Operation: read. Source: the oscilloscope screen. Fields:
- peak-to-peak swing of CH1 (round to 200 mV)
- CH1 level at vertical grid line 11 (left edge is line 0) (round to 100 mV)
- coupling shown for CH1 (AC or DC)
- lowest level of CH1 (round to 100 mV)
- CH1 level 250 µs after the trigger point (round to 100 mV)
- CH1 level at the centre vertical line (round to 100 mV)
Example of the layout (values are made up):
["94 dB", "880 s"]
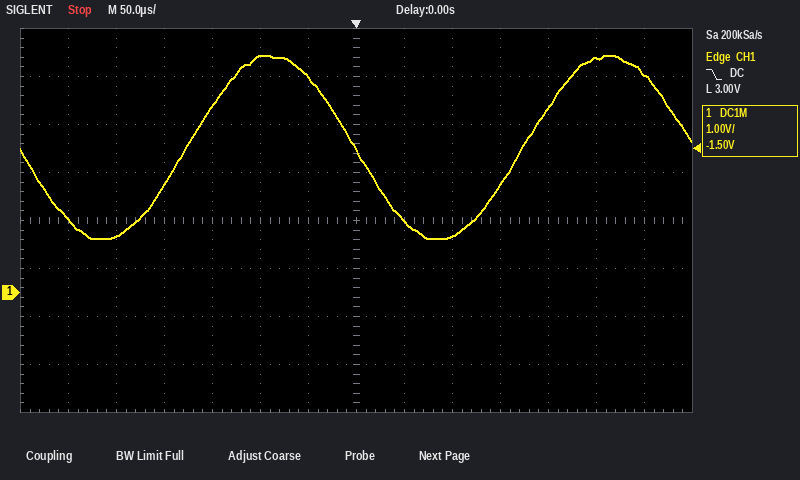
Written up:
["3.8 V", "3.8 V", "DC", "1.1 V", "4.9 V", "3.0 V"]
